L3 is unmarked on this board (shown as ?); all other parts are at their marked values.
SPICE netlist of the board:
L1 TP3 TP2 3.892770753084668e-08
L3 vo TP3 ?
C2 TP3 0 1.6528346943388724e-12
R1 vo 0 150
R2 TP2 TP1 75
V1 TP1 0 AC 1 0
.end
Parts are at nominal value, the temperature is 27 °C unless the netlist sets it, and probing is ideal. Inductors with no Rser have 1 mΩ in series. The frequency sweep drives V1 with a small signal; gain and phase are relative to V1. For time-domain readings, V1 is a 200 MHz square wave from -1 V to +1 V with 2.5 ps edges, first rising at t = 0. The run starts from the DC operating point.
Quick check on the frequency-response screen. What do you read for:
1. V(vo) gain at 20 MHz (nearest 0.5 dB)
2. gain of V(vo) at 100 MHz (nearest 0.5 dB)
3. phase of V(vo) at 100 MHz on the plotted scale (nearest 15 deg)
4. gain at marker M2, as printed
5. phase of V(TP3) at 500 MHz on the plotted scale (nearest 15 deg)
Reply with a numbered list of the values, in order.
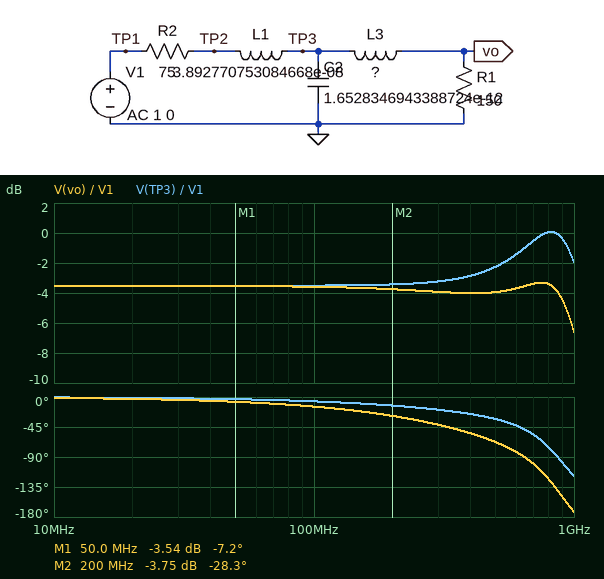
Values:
1. -3.5 dB
2. -3.5 dB
3. -15 deg
4. -3.75 dB
5. -30 deg
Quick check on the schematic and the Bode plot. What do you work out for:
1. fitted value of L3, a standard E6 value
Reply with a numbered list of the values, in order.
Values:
1. 33 nH
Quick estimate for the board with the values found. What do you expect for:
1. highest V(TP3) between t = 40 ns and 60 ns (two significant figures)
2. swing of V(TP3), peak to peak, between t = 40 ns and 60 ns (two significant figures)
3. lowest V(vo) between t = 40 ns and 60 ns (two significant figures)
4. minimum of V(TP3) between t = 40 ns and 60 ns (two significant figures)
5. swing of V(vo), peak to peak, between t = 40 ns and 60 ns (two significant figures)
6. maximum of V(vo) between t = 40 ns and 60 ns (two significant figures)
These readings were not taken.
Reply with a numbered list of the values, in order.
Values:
1. 1.0 V
2. 2.0 V
3. -790 mV
4. -1.0 V
5. 1.6 V
6. 790 mV
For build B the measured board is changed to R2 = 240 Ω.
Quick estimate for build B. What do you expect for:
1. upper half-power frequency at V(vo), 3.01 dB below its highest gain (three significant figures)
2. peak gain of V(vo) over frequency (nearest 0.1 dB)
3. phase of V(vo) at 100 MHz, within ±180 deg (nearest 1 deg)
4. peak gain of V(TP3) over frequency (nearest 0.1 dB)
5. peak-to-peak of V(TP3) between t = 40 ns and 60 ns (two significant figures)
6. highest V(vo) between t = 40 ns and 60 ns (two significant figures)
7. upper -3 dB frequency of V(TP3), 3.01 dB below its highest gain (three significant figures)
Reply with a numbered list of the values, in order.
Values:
1. 958 MHz
2. -8.2 dB
3. -12 deg
4. -5.6 dB
5. 1.2 V
6. 460 mV
7. 1.11 GHz
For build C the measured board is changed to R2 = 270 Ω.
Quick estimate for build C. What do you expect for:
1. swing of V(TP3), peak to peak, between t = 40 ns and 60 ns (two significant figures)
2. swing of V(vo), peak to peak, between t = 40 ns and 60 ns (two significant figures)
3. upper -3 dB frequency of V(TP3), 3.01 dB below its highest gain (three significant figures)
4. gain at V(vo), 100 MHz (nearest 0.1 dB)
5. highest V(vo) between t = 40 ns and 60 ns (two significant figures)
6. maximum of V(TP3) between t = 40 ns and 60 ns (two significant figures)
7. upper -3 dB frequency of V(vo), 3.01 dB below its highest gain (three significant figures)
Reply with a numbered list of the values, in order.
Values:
1. 1.1 V
2. 860 mV
3. 1.11 GHz
4. -8.9 dB
5. 430 mV
6. 540 mV
7. 946 MHz
